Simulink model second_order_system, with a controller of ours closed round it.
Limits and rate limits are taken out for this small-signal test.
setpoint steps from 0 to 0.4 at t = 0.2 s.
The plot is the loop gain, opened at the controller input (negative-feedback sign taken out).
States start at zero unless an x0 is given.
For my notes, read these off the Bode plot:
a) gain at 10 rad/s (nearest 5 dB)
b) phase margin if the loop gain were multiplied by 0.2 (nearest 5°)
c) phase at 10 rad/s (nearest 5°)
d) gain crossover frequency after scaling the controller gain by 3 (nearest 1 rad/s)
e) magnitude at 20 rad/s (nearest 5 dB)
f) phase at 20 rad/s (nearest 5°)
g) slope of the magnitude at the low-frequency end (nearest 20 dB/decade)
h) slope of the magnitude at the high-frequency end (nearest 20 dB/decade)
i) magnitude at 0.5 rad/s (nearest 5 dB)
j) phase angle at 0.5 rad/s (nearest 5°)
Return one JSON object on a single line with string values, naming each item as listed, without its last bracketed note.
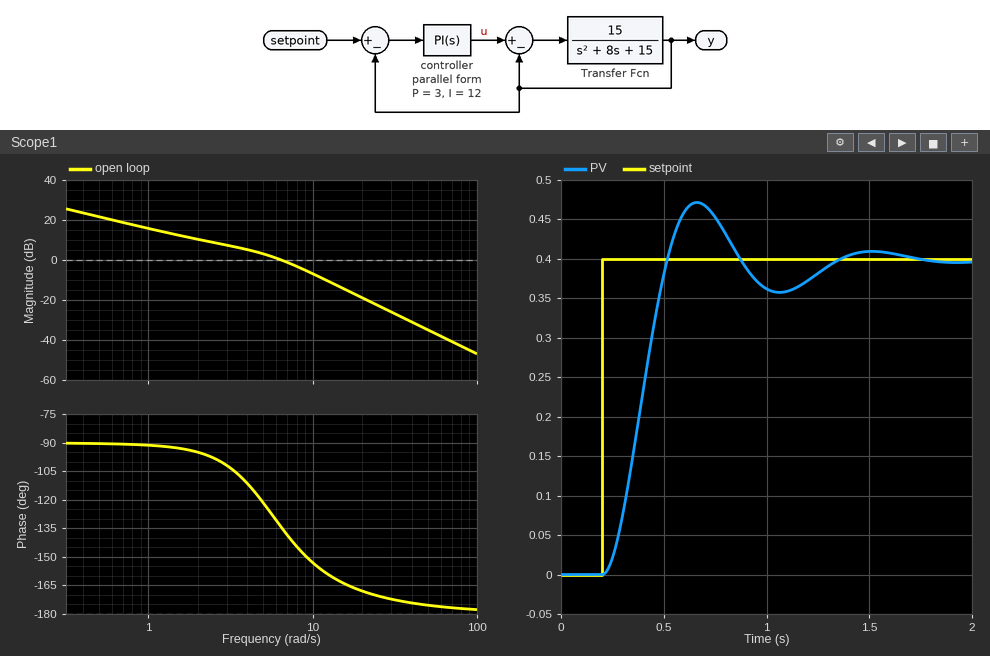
{"gain at 10 rad/s": "-5 dB", "phase margin if the loop gain were multiplied by 0.2": "90°", "phase at 10 rad/s": "-155°", "gain crossover frequency after scaling the controller gain by 3": "12 rad/s", "magnitude at 20 rad/s": "-20 dB", "phase at 20 rad/s": "-170°", "slope of the magnitude at the low-frequency end": "-20 dB/decade", "slope of the magnitude at the high-frequency end": "-40 dB/decade", "magnitude at 0.5 rad/s": "20 dB", "phase angle at 0.5 rad/s": "-90°"}
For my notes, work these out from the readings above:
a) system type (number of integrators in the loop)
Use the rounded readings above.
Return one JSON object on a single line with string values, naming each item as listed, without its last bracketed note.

{"system type": "1"}
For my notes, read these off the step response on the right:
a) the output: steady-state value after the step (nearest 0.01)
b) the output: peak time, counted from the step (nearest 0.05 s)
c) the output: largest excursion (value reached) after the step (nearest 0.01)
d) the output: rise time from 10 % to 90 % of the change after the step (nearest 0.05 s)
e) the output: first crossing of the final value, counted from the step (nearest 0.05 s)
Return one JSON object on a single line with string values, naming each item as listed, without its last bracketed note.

{"the output: steady-state value after the step": "0.40", "the output: peak time, counted from the step": "0.45 s", "the output: largest excursion (value reached) after the step": "0.47", "the output: rise time from 10 % to 90 % of the change after the step": "0.20 s", "the output: first crossing of the final value, counted from the step": "0.30 s"}
